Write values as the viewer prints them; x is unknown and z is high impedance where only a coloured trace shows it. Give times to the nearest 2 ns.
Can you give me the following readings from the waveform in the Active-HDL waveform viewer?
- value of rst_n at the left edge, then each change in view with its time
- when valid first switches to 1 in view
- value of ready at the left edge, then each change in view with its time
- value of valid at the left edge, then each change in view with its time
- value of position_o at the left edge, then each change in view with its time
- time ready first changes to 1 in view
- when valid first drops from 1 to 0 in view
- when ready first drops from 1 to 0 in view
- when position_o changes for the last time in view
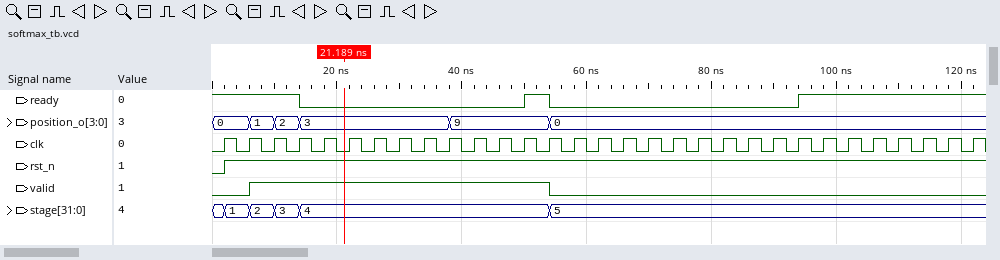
0, 1 at 2 ns
6 ns
1, 0 at 14 ns, 1 at 50 ns, 0 at 54 ns, 1 at 94 ns
0, 1 at 6 ns, 0 at 54 ns
0, 1 at 6 ns, 2 at 10 ns, 3 at 14 ns, 9 at 38 ns, 0 at 54 ns
50 ns
54 ns
14 ns
54 ns
